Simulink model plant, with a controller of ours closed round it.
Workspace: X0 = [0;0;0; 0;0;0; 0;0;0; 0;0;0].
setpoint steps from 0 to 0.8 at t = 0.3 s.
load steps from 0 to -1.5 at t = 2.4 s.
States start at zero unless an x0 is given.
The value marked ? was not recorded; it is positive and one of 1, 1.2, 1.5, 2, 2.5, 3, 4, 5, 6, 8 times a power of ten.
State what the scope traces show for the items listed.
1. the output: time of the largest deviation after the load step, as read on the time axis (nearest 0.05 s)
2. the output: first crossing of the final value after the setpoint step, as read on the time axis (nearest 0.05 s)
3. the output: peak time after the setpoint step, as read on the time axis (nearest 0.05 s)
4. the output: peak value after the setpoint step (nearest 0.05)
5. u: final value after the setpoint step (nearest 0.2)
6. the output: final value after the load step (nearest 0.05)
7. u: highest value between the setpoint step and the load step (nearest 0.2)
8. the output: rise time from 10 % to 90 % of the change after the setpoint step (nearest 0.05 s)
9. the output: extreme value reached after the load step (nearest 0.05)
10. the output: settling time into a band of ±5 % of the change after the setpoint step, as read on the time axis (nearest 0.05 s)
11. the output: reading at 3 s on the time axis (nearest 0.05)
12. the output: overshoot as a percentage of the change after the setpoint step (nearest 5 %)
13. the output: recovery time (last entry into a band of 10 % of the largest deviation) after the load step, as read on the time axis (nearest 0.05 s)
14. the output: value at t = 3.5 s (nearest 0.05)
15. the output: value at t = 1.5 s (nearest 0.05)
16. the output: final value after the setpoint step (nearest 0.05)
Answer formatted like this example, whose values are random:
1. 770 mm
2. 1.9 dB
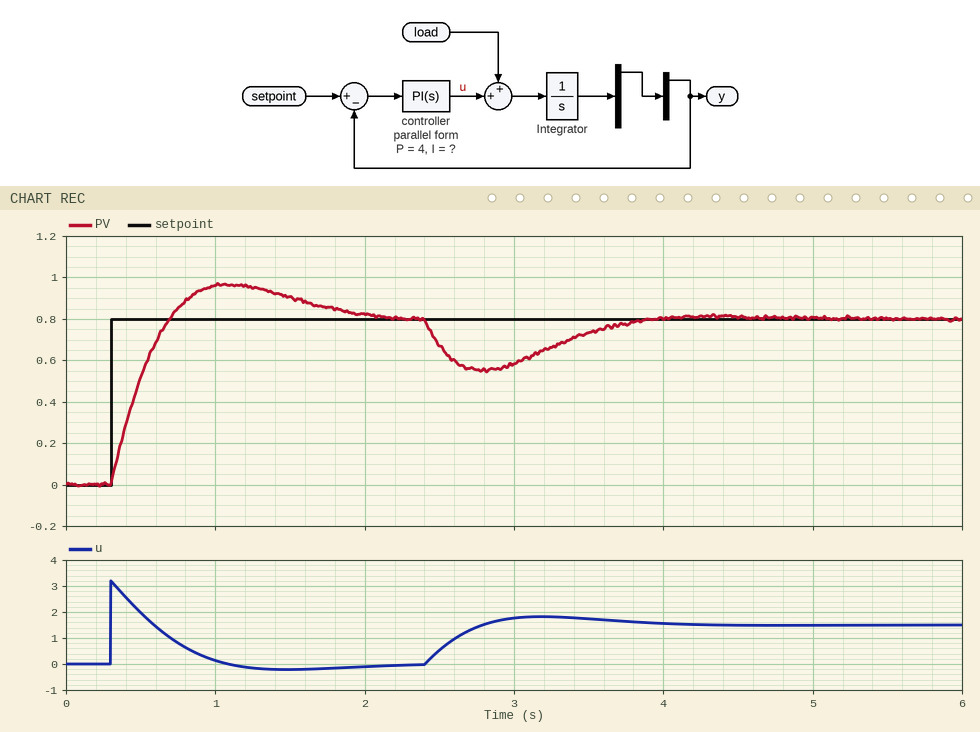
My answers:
1. 2.80 s
2. 0.70 s
3. 1.10 s
4. 0.95
5. 0.0
6. 0.80
7. 3.2
8. 0.30 s
9. 0.55
10. 1.85 s
11. 0.60
12. 20 %
13. 3.75 s
14. 0.75
15. 0.90
16. 0.80
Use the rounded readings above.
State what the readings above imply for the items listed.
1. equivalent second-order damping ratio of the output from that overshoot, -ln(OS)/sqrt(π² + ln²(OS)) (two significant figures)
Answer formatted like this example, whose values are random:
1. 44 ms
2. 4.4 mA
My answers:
1. 0.46
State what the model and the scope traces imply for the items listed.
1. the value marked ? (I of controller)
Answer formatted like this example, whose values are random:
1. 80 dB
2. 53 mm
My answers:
1. 8
